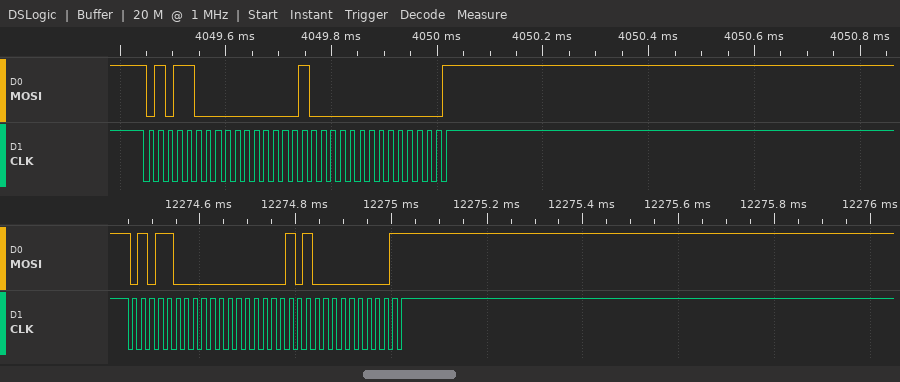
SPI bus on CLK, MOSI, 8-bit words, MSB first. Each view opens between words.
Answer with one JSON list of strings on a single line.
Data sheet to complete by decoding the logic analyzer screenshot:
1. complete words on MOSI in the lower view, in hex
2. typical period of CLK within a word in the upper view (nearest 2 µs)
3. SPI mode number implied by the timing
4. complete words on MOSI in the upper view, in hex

["58, 00, 28, 03", "18 µs", "3", "58, 00, 80, 01"]
